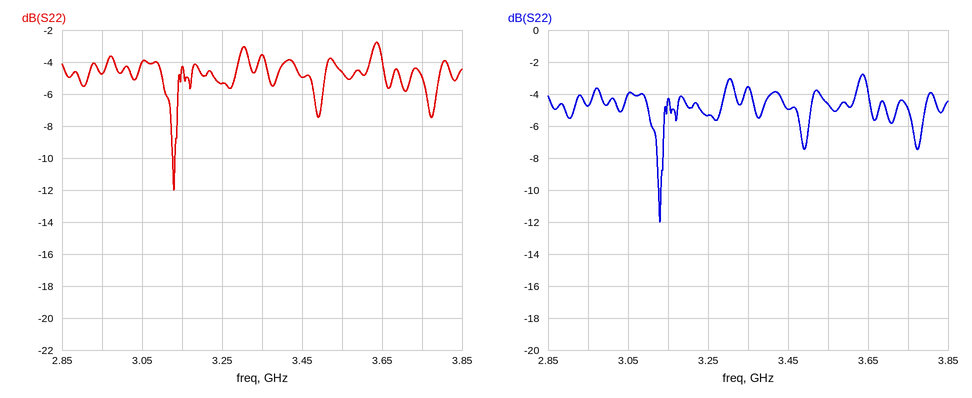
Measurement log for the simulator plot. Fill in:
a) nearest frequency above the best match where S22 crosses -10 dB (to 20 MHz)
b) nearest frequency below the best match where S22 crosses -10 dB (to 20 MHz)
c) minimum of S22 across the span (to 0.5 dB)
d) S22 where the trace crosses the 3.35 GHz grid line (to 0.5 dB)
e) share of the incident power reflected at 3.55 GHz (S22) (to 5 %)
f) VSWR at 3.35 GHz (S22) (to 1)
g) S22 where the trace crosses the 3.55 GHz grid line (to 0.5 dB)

3.14 GHz
3.12 GHz
-12.0 dB
-3.5 dB
35 %
5
-4.5 dB
